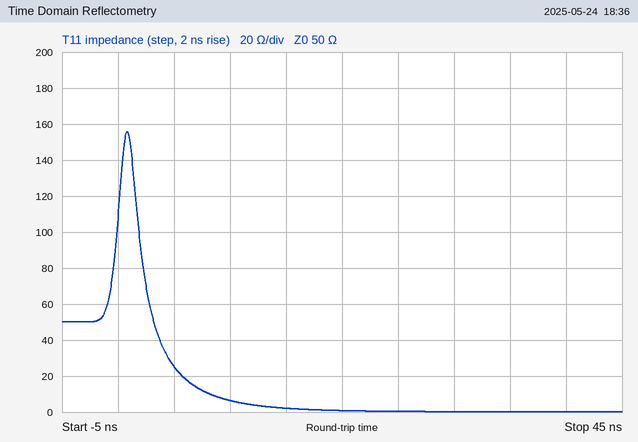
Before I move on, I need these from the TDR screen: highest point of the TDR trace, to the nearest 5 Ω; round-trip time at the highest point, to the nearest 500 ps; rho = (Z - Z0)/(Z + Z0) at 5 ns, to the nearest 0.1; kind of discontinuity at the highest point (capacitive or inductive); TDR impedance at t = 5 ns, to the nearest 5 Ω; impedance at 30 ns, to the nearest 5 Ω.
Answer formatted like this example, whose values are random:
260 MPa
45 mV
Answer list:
155 Ω
1.0 ns
-0.3
inductive
25 Ω
0 Ω
